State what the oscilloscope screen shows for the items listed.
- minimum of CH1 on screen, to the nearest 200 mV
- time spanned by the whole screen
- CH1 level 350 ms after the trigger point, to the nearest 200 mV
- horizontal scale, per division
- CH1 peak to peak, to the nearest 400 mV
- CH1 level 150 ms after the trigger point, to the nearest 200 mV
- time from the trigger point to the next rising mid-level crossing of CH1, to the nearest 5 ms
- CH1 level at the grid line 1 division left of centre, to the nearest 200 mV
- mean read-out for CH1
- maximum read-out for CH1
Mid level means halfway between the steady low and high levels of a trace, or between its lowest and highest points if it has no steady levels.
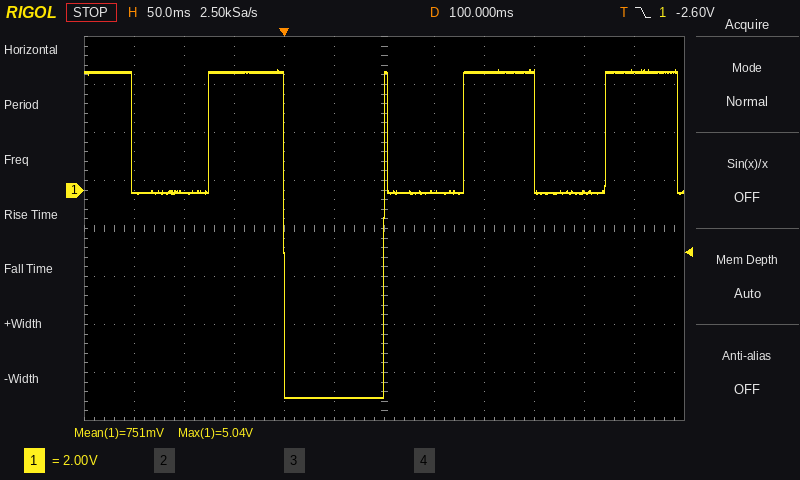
-8.6 V
600 ms
5.0 V
50 ms
13.6 V
0.0 V
100 ms
-8.6 V
751 mV
5.04 V
